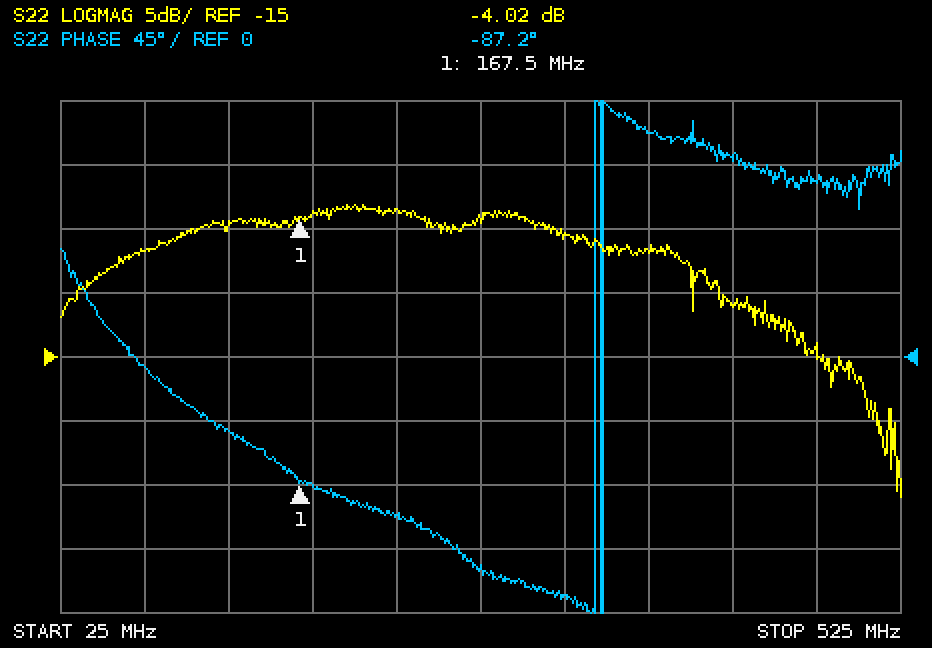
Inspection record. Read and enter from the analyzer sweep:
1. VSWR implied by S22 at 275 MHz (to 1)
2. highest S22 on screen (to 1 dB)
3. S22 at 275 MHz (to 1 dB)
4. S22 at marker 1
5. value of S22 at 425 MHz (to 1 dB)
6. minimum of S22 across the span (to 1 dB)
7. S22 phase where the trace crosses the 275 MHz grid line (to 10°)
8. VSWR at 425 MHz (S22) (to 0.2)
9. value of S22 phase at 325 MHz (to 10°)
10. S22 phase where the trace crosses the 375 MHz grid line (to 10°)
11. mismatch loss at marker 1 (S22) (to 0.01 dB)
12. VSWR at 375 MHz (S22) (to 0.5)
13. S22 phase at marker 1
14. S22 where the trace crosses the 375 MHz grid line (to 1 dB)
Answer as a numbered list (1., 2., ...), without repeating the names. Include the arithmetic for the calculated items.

1. |Γ| = 10^(-4/20) = 0.6310; VSWR = (1 + 0.6310)/(1 − 0.6310) ≈ 4
2. -3 dB
3. -4 dB
4. -4.02 dB
5. -11 dB
6. -26 dB
7. -150°
8. |Γ| = 10^(-11/20) = 0.2818; VSWR = (1 + 0.2818)/(1 − 0.2818) ≈ 1.8
9. -170°
10. 160°
11. −10 log10(1 − 10^(-4.02/10)) ≈ 2.19 dB
12. |Γ| = 10^(-7/20) = 0.4467; VSWR = (1 + 0.4467)/(1 − 0.4467) ≈ 2.61, so 2.5 to the nearest 0.5
13. -87.2°
14. -7 dB
